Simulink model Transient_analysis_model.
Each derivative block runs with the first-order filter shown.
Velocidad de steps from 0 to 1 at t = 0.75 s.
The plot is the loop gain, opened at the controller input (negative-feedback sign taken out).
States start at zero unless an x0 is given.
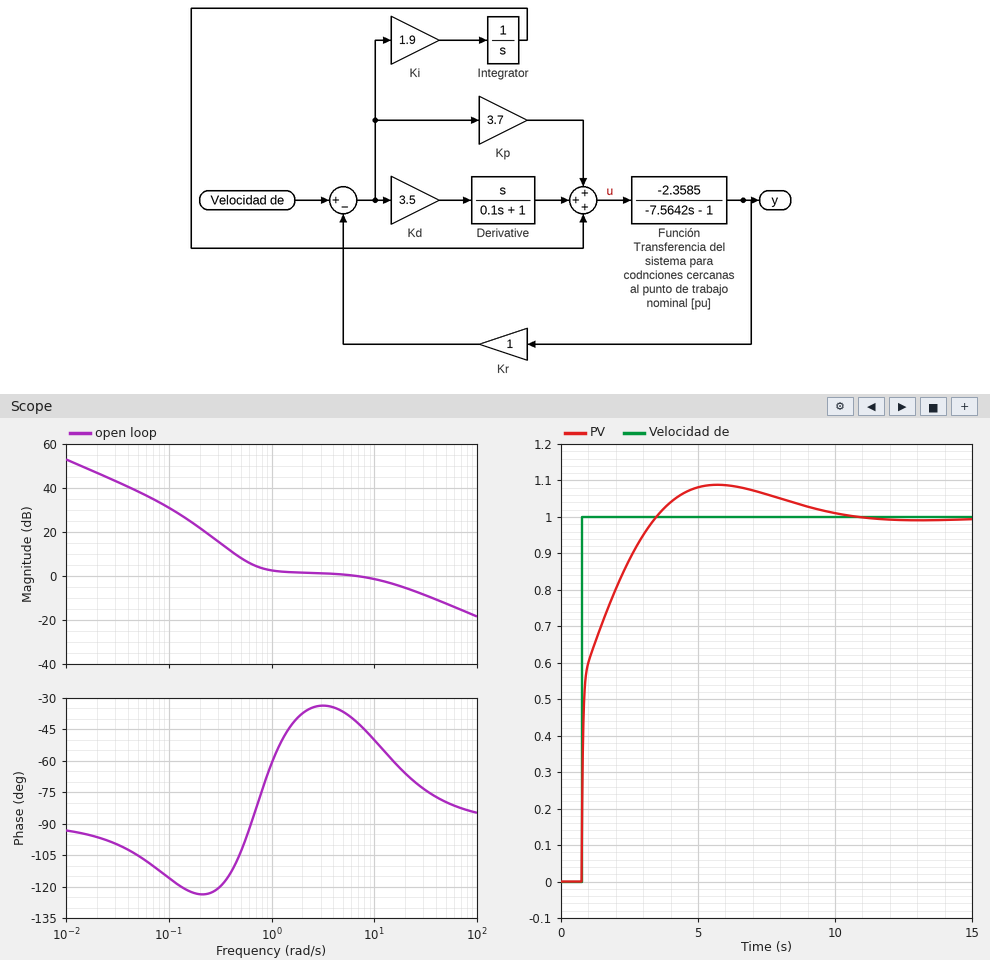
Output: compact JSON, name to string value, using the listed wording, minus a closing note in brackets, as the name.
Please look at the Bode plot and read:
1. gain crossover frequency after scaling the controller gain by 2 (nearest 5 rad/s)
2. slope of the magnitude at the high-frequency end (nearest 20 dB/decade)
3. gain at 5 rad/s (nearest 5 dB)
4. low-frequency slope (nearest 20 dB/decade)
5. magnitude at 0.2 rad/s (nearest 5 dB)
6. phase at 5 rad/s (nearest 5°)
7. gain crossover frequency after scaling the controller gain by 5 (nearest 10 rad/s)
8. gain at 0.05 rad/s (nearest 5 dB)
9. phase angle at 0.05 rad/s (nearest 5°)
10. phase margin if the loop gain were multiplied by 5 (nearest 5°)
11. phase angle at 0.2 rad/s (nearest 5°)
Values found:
{"gain crossover frequency after scaling the controller gain by 2": "20 rad/s", "slope of the magnitude at the high-frequency end": "-20 dB/decade", "gain at 5 rad/s": "0 dB", "low-frequency slope": "-20 dB/decade", "magnitude at 0.2 rad/s": "20 dB", "phase at 5 rad/s": "-35°", "gain crossover frequency after scaling the controller gain by 5": "60 rad/s", "gain at 0.05 rad/s": "40 dB", "phase angle at 0.05 rad/s": "-105°", "phase margin if the loop gain were multiplied by 5": "100°", "phase angle at 0.2 rad/s": "-125°"}
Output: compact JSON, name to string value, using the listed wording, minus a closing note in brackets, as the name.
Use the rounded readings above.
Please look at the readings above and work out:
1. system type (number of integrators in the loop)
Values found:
{"system type": "1"}
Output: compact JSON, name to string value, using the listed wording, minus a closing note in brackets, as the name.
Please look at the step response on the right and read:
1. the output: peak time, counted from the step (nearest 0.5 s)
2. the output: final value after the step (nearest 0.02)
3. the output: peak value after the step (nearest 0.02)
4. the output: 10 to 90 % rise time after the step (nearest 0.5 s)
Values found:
{"the output: peak time, counted from the step": "5.0 s", "the output: final value after the step": "1.00", "the output: peak value after the step": "1.08", "the output: 10 to 90 % rise time after the step": "2.0 s"}
